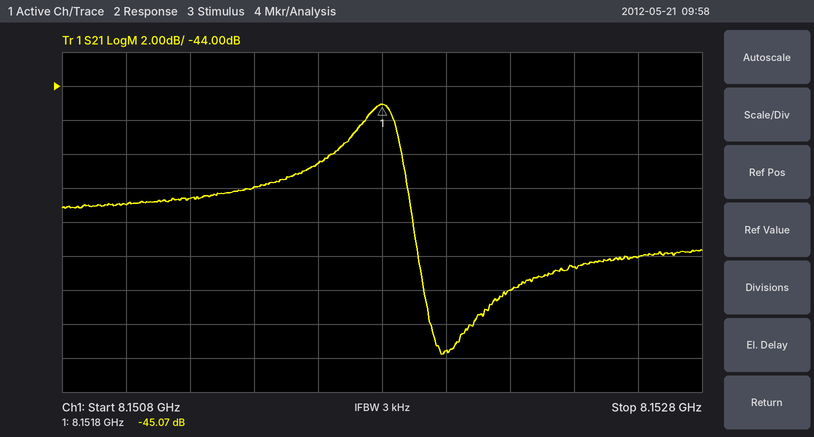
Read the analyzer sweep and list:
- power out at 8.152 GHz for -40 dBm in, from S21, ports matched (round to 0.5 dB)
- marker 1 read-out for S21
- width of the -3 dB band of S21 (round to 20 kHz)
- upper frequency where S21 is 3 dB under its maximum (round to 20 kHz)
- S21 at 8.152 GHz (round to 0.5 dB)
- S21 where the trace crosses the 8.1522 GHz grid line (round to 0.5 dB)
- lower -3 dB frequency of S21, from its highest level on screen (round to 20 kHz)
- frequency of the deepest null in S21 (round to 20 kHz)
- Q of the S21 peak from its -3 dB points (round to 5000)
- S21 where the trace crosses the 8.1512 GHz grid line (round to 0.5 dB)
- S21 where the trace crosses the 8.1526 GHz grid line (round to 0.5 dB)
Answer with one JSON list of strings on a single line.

["-99.5 dBm", "-45.07 dB", "220 kHz", "8.15186 GHz", "-59.5 dB", "-56.0 dB", "8.15164 GHz", "8.15198 GHz", "35000", "-50.5 dB", "-54.0 dB"]
